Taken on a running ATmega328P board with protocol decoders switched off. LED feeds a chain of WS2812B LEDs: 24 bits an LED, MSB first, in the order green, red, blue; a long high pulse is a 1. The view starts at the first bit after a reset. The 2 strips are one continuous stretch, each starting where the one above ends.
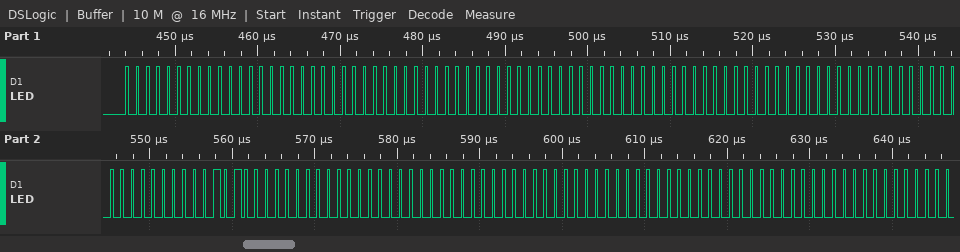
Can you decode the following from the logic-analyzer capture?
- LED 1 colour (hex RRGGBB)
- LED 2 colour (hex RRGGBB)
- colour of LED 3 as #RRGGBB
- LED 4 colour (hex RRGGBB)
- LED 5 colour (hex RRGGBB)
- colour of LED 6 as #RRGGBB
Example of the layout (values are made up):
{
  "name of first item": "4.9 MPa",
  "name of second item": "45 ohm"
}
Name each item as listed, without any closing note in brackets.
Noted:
{
  "LED 1 colour": "#000000",
  "LED 2 colour": "#000000",
  "colour of LED 3 as #RRGGBB": "#000000",
  "LED 4 colour": "#000014",
  "LED 5 colour": "#000000",
  "colour of LED 6 as #RRGGBB": "#000000"
}
